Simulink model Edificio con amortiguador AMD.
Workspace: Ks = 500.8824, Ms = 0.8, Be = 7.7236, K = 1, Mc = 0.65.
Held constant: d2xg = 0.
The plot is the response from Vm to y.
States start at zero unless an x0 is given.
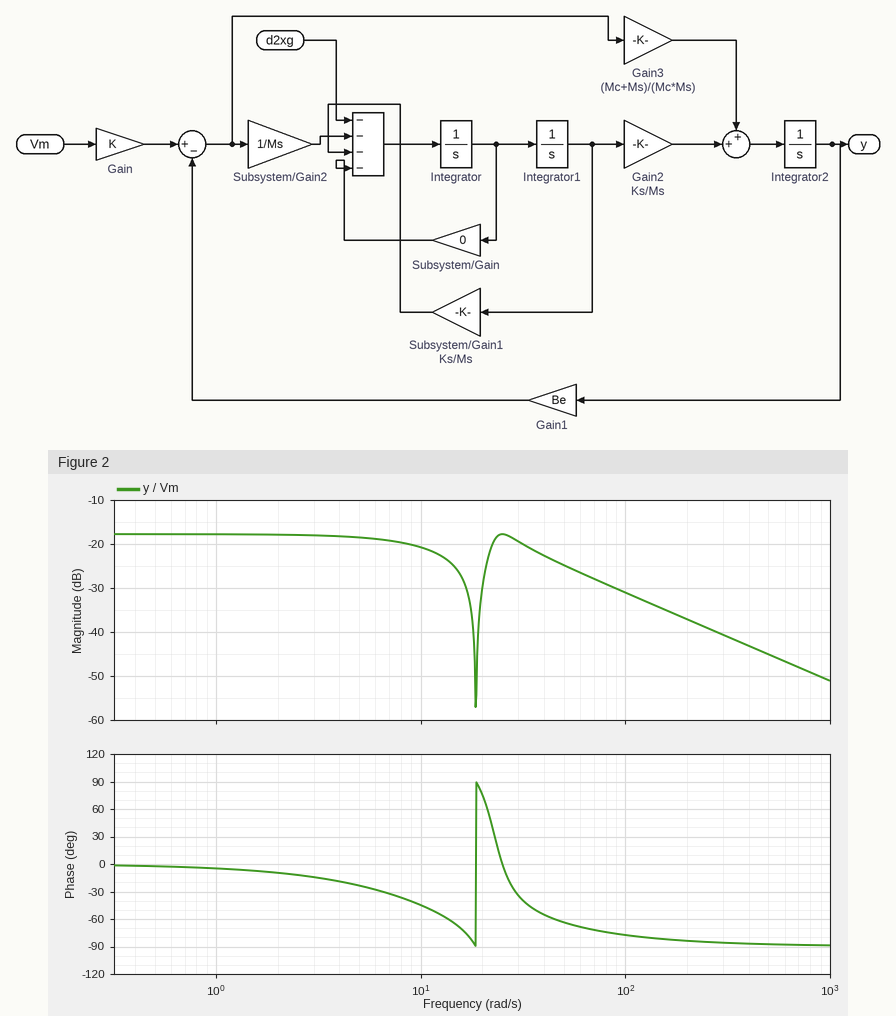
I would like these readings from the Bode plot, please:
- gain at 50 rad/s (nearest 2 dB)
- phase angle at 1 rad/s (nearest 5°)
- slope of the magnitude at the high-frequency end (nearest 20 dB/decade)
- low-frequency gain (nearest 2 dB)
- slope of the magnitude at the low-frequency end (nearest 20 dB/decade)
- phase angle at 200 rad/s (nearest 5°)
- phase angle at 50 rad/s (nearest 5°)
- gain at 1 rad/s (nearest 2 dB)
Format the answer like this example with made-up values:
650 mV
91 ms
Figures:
-24 dB
-5°
-20 dB/decade
-18 dB
0 dB/decade
-85°
-65°
-18 dB
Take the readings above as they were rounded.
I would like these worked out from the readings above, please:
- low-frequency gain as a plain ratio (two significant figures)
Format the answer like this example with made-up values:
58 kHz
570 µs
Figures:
0.13
